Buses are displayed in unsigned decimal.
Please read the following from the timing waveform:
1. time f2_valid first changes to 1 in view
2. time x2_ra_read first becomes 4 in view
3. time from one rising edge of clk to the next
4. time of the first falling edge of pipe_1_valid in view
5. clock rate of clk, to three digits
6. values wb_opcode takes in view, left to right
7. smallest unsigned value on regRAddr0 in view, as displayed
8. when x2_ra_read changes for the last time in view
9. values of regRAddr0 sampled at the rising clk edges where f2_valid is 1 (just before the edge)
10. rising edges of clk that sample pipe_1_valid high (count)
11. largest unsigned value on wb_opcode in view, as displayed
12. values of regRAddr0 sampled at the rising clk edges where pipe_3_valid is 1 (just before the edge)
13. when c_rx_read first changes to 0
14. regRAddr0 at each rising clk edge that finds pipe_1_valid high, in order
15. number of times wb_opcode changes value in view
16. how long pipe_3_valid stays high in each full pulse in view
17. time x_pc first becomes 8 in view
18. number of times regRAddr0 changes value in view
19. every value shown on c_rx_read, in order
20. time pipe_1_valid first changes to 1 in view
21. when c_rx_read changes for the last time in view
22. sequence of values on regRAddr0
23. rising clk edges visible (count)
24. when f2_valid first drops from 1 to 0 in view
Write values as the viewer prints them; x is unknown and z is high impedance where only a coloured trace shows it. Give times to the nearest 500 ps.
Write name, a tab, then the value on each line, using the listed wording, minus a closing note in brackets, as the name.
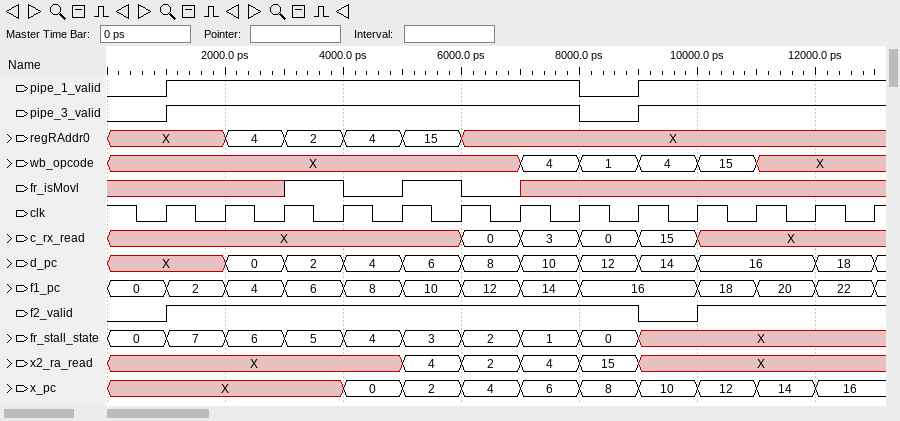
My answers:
time f2_valid first changes to 1 in view	1000 ps
time x2_ra_read first becomes 4 in view	5000 ps
time from one rising edge of clk to the next	1000 ps
time of the first falling edge of pipe_1_valid in view	8000 ps
clock rate of clk, to three digits	1.00 GHz
values wb_opcode takes in view, left to right	X, 4, 1, 4, 15, X
smallest unsigned value on regRAddr0 in view, as displayed	2
when x2_ra_read changes for the last time in view	9000 ps
values of regRAddr0 sampled at the rising clk edges where f2_valid is 1	X, 4, 2, 4, 15, X, X, X, X, X, X
rising edges of clk that sample pipe_1_valid high	11
largest unsigned value on wb_opcode in view, as displayed	15
values of regRAddr0 sampled at the rising clk edges where pipe_3_valid is 1	X, 4, 2, 4, 15, X, X, X, X, X, X
when c_rx_read first changes to 0	6000 ps
regRAddr0 at each rising clk edge that finds pipe_1_valid high, in order	X, 4, 2, 4, 15, X, X, X, X, X, X
number of times wb_opcode changes value in view	5
how long pipe_3_valid stays high in each full pulse in view	7000 ps
time x_pc first becomes 8 in view	8000 ps
number of times regRAddr0 changes value in view	5
every value shown on c_rx_read, in order	X, 0, 3, 0, 15, X
time pipe_1_valid first changes to 1 in view	1000 ps
when c_rx_read changes for the last time in view	10000 ps
sequence of values on regRAddr0	X, 4, 2, 4, 15, X
rising clk edges visible	13
when f2_valid first drops from 1 to 0 in view	9000 ps
